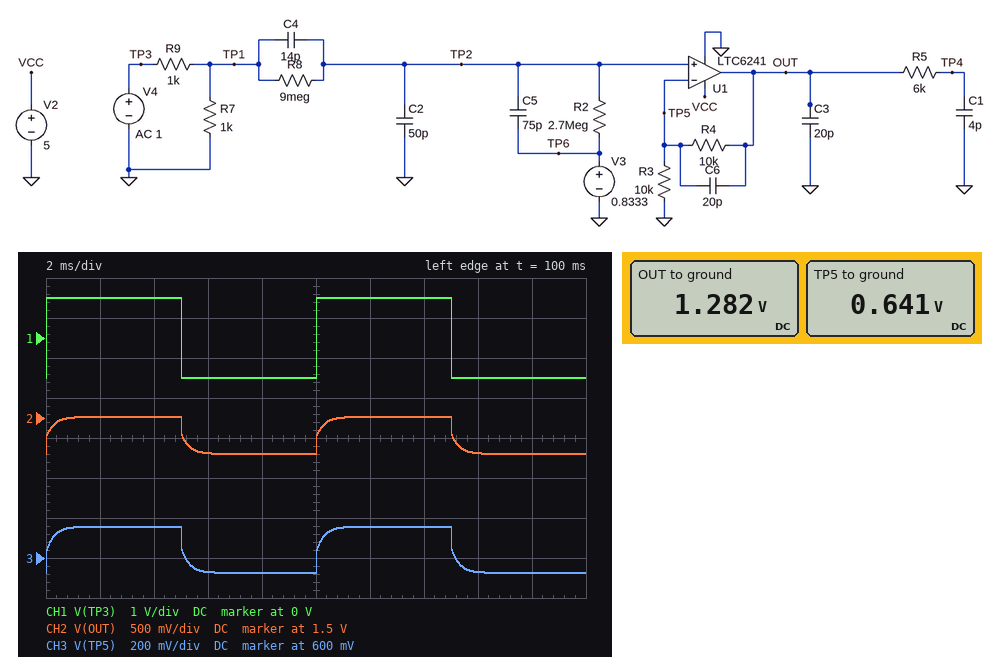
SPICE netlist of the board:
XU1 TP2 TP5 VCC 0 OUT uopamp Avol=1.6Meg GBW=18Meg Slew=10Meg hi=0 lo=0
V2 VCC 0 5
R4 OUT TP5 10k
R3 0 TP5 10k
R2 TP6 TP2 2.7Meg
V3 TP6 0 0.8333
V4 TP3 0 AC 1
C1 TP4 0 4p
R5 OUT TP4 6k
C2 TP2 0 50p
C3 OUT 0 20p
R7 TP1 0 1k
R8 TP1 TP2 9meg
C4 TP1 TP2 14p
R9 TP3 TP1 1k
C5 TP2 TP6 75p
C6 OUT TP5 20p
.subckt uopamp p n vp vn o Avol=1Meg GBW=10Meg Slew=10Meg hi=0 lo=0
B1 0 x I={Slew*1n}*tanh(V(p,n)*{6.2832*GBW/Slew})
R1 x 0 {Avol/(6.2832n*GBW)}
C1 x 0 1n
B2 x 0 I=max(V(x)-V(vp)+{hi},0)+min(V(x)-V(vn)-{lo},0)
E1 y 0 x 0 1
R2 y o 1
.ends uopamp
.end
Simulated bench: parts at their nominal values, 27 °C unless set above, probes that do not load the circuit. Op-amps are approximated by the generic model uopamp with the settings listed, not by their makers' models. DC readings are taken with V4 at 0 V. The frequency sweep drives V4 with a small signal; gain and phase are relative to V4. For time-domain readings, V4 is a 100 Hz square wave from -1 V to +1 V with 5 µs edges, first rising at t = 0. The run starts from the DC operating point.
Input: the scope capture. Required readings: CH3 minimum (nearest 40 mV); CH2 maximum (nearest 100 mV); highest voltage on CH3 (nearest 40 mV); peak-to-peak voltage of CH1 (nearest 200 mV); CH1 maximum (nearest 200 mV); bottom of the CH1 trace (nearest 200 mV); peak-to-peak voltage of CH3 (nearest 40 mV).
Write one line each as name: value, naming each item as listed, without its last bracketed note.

CH3 minimum: 520 mV
CH2 maximum: 1.5 V
highest voltage on CH3: 760 mV
peak-to-peak voltage of CH1: 2.0 V
CH1 maximum: 1.0 V
bottom of the CH1 trace: -1.0 V
peak-to-peak voltage of CH3: 240 mV
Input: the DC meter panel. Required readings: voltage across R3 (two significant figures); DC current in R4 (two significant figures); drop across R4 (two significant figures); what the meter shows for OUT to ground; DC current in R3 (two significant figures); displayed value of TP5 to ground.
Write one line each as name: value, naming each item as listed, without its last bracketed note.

voltage across R3: 640 mV
DC current in R4: 64 µA
drop across R4: 640 mV
what the meter shows for OUT to ground: 1.282 V
DC current in R3: 64 µA
displayed value of TP5 to ground: 0.641 V
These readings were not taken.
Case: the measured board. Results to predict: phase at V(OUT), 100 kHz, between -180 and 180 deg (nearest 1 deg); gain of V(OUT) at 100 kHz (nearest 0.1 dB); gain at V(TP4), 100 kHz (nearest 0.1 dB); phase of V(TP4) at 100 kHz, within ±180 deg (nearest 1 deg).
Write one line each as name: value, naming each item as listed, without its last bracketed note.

phase at V(OUT), 100 kHz, between -180 and 180 deg: -5 deg
gain of V(OUT) at 100 kHz: -20.0 dB
gain at V(TP4), 100 kHz: -20.0 dB
phase of V(TP4) at 100 kHz, within ±180 deg: -6 deg
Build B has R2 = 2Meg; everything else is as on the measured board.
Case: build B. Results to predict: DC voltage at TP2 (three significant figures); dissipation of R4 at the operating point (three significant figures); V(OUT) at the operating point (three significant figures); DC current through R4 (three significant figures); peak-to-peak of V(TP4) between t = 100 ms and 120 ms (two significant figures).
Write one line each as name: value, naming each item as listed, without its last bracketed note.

DC voltage at TP2: 682 mV
dissipation of R4 at the operating point: 46.5 µW
V(OUT) at the operating point: 1.36 V
DC current through R4: 68.2 µA
peak-to-peak of V(TP4) between t = 100 ms and 120 ms: 360 mV
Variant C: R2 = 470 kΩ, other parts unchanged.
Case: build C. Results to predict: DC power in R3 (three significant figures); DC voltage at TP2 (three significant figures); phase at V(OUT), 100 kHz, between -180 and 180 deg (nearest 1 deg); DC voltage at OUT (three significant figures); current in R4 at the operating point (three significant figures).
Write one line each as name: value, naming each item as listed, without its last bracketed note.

DC power in R3: 62.7 µW
DC voltage at TP2: 792 mV
phase at V(OUT), 100 kHz, between -180 and 180 deg: -4 deg
DC voltage at OUT: 1.58 V
current in R4 at the operating point: 79.2 µA
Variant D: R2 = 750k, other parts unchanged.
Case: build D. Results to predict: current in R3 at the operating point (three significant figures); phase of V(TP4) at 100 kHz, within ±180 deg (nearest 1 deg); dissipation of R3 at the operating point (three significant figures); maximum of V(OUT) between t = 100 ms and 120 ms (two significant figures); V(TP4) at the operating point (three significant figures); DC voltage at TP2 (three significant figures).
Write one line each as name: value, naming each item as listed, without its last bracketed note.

current in R3 at the operating point: 76.9 µA
phase of V(TP4) at 100 kHz, within ±180 deg: -5 deg
dissipation of R3 at the operating point: 59.2 µW
maximum of V(OUT) between t = 100 ms and 120 ms: 1.7 V
V(TP4) at the operating point: 1.54 V
DC voltage at TP2: 769 mV
